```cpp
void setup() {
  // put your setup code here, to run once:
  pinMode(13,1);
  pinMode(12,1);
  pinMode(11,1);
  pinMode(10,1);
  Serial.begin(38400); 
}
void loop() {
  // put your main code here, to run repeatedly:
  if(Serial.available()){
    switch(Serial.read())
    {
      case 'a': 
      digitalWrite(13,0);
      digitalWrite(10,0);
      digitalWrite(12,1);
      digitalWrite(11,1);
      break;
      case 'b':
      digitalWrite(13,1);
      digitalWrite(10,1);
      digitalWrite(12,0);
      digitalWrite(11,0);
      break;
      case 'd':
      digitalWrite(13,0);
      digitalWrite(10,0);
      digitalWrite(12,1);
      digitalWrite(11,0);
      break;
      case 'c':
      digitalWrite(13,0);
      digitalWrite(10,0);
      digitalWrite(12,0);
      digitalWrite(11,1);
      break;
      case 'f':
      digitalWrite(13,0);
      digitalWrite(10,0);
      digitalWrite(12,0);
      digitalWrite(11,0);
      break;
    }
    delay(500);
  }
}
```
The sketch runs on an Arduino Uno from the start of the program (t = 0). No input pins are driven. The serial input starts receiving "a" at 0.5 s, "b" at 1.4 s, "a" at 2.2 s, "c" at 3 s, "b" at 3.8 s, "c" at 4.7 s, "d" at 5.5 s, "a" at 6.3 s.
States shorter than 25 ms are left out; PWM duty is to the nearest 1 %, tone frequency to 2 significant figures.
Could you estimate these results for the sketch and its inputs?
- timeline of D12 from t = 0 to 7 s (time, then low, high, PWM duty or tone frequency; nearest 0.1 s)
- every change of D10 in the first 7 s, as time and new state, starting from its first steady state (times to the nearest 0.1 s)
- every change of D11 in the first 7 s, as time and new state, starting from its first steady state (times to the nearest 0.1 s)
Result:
0 s low; 0.5 s high; 1.4 s low; 2.2 s high; 3 s low; 5.5 s high
0 s low; 1.4 s high; 2.2 s low; 3.8 s high; 4.7 s low
0 s low; 0.5 s high; 1.4 s low; 2.2 s high; 3.8 s low; 4.7 s high; 5.5 s low; 6.3 s high
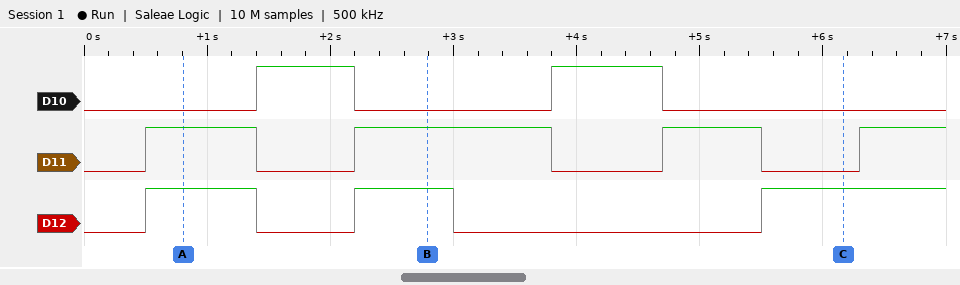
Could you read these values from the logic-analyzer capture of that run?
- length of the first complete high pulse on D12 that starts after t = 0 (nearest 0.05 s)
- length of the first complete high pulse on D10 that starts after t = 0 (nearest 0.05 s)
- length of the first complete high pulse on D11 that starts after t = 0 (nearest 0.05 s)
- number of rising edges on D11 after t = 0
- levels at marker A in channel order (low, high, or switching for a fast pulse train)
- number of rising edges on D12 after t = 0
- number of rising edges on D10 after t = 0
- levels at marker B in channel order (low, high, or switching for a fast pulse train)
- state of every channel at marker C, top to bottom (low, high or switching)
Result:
0.90 s
0.80 s
0.90 s
4
D10 low, D11 high, D12 high
3
2
D10 low, D11 high, D12 high
D10 low, D11 low, D12 high
